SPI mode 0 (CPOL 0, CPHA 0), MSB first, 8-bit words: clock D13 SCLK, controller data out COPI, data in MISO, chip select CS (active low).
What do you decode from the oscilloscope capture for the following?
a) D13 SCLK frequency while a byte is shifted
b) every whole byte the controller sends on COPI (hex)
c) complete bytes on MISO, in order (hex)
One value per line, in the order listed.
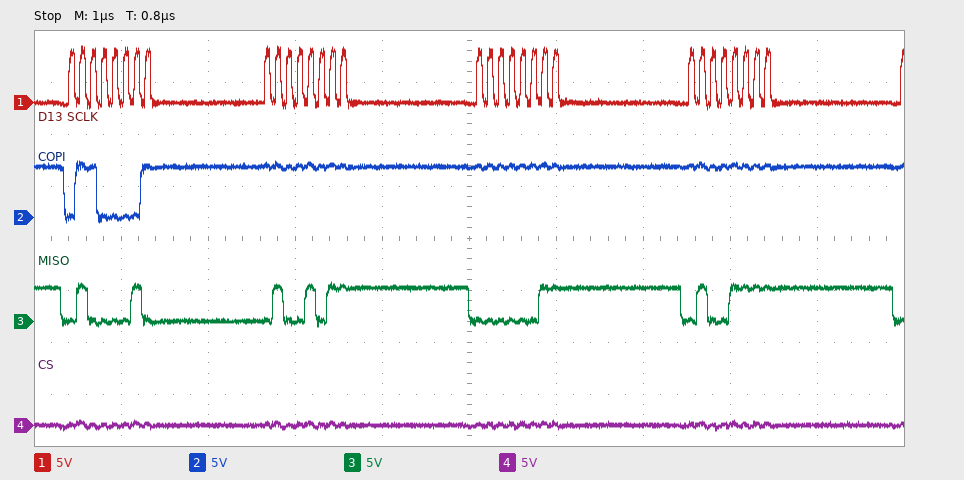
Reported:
8 MHz
61 FF FF FF
42 4B 03 4F
